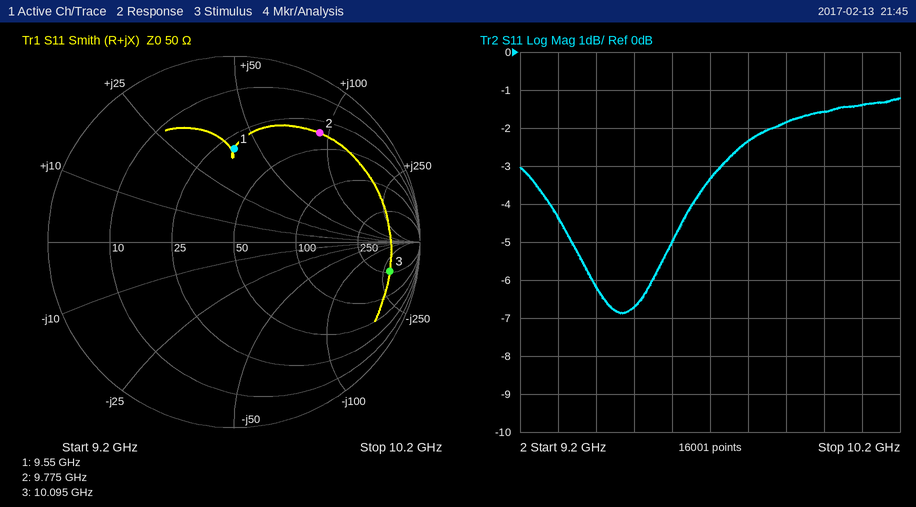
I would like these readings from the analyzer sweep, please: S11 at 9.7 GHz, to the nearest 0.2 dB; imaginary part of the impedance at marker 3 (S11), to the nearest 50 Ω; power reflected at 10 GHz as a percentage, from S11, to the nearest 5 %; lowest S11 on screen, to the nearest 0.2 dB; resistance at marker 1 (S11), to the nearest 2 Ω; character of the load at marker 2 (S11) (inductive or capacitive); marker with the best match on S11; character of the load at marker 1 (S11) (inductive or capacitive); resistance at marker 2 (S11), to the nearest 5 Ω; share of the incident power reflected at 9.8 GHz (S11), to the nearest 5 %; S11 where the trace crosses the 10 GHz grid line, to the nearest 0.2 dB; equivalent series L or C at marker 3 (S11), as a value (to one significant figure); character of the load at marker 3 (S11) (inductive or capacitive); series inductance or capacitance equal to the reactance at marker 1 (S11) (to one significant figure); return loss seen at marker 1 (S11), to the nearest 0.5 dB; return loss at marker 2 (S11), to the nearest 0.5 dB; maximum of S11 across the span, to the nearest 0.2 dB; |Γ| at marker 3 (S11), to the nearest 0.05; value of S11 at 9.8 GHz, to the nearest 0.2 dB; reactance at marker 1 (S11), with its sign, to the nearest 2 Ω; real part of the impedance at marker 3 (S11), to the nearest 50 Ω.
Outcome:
-3.4 dB
-300 Ω
70 %
-6.8 dB
30 Ω
inductive
marker 1
inductive
35 Ω
60 %
-1.6 dB
50 fF
capacitive
700 pH
6.0 dB
2.5 dB
-1.2 dB
0.85
-2.4 dB
+40 Ω
250 Ω
